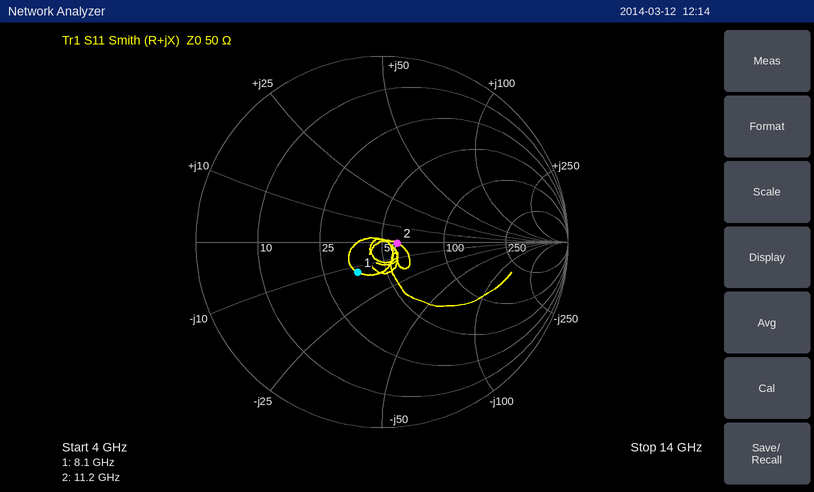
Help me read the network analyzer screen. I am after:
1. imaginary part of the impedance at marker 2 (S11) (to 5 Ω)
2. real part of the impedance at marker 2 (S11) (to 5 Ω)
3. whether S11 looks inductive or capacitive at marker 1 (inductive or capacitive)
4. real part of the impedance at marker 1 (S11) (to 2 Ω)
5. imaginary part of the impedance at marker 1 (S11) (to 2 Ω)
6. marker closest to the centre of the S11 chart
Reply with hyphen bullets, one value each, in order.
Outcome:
- 0 Ω
- 60 Ω
- capacitive
- 36 Ω
- -12 Ω
- marker 2
